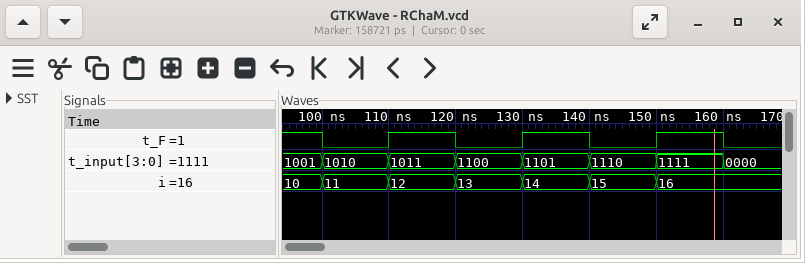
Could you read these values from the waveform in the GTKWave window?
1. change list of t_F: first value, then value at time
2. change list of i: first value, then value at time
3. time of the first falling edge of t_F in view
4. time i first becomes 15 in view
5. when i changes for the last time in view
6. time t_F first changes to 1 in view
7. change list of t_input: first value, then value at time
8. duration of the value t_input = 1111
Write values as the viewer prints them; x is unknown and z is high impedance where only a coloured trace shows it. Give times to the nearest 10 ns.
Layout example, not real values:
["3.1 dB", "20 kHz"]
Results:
["1, 0 at 100 ns, 1 at 110 ns, 0 at 120 ns, 1 at 130 ns, 0 at 140 ns, 1 at 150 ns, 0 at 160 ns", "10, 11 at 100 ns, 12 at 110 ns, 13 at 120 ns, 14 at 130 ns, 15 at 140 ns, 16 at 150 ns", "100 ns", "140 ns", "150 ns", "110 ns", "1001, 1010 at 100 ns, 1011 at 110 ns, 1100 at 120 ns, 1101 at 130 ns, 1110 at 140 ns, 1111 at 150 ns, 0000 at 160 ns", "10 ns"]
